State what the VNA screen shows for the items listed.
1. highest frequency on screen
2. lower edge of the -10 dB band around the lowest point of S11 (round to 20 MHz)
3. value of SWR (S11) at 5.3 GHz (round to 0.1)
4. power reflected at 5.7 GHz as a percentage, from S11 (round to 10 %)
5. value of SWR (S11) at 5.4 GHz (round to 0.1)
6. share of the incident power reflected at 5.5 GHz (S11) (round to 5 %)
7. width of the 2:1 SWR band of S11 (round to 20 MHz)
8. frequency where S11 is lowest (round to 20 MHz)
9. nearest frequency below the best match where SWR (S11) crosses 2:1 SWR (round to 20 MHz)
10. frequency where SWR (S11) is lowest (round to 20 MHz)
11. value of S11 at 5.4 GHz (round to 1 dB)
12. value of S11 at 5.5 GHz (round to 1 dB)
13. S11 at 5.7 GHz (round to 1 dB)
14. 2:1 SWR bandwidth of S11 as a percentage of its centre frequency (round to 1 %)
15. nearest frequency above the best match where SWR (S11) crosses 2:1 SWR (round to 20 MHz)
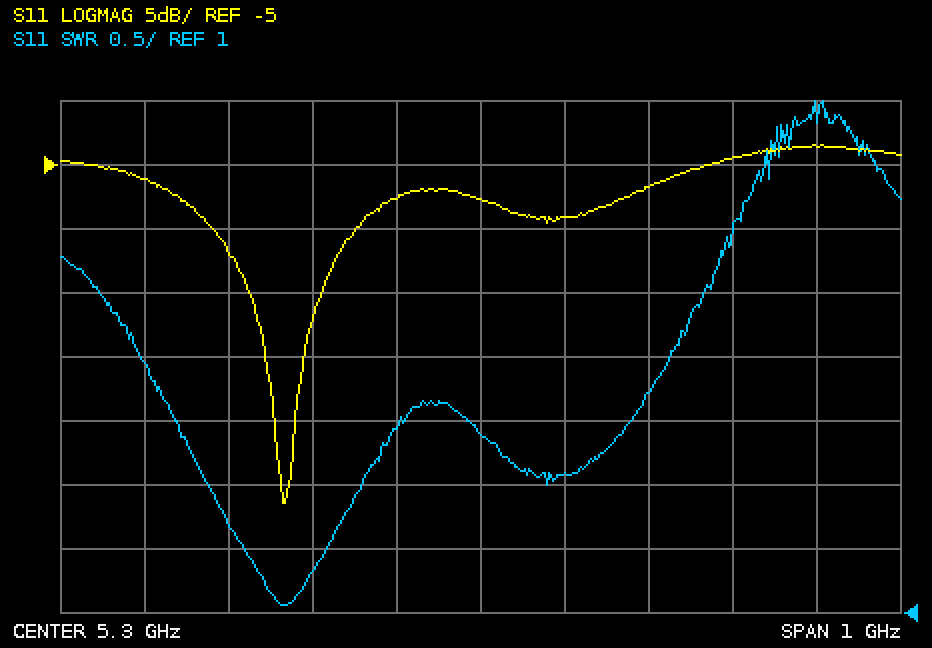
5.8 GHz
4.98 GHz
2.4
40 %
2.1
20 %
180 MHz
5.06 GHz
4.98 GHz
5.06 GHz
-9 dB
-7 dB
-4 dB
4 %
5.16 GHz
